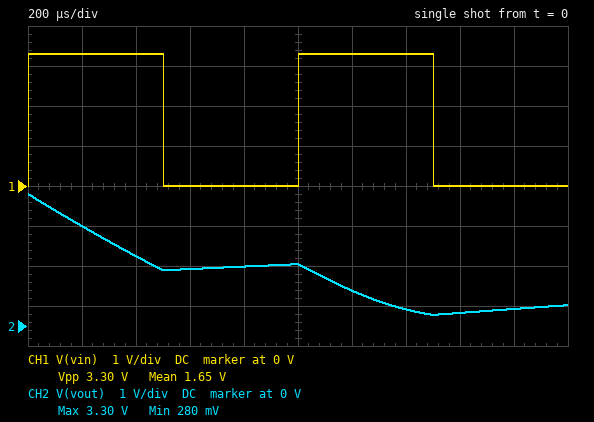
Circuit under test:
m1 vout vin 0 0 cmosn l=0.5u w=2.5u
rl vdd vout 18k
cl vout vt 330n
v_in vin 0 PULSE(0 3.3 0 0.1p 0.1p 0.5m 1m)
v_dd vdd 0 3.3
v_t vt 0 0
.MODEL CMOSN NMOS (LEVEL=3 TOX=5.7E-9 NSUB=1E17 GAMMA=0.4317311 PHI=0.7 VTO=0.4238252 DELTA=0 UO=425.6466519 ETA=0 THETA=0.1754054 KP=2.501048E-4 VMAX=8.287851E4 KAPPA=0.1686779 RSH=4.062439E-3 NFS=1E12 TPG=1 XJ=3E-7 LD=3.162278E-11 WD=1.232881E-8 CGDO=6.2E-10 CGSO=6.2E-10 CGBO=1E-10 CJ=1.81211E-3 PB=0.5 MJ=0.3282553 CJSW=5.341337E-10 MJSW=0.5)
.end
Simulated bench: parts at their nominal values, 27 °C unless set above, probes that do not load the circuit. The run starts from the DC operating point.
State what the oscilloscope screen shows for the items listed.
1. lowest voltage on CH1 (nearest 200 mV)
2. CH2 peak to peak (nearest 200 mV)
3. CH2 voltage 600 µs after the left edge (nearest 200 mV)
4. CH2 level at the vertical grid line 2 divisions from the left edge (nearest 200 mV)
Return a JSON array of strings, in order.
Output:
["0 V", "3.0 V", "1.4 V", "1.8 V"]
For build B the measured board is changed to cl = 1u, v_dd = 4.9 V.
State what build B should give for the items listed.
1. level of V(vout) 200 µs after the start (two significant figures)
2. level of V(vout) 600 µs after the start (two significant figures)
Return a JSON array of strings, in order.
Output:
["4.6 V", "4.2 V"]
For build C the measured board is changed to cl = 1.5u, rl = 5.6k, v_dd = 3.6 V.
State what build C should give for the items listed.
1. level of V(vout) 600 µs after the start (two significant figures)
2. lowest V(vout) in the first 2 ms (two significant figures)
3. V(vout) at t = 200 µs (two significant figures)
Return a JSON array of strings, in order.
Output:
["3.2 V", "2.8 V", "3.4 V"]
